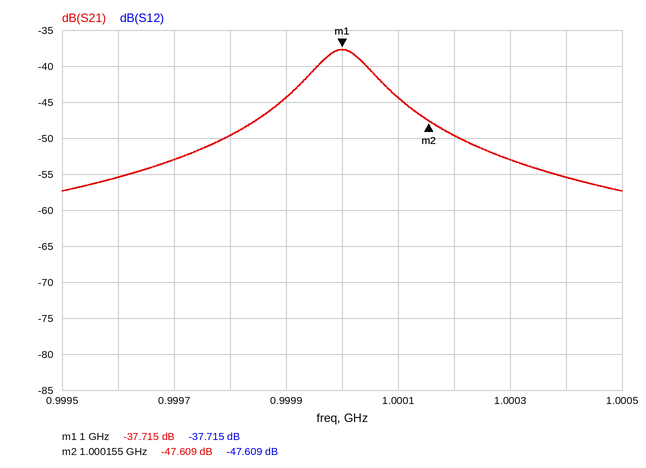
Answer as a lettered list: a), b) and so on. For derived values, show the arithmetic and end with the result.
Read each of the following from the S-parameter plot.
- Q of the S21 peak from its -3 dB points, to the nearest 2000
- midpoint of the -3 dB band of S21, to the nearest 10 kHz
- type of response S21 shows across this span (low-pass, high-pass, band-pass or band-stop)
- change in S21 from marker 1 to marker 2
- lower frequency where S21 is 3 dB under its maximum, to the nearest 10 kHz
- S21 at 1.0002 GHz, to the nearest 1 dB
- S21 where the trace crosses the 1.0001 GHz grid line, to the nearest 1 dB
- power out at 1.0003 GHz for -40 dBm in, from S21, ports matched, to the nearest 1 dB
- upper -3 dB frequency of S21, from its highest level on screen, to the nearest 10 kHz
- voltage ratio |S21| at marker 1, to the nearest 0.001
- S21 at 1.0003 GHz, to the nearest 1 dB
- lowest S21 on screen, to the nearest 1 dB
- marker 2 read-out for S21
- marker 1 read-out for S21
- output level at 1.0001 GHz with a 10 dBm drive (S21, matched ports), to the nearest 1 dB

a) 1 GHz / 100 kHz ≈ 10000
b) 1.00000 GHz
c) band-pass
d) -47.609 − (-37.715) = -9.894 dB
e) 999.95 MHz
f) -50 dB
g) -44 dB
h) -40 dBm + (-53 dB) = -93 dBm
i) 1.00005 GHz
j) 10^(-37.715/20) ≈ 0.013
k) -53 dB
l) -57 dB
m) -47.609 dB
n) -37.715 dB
o) 10 dBm + (-44 dB) = -34 dBm
